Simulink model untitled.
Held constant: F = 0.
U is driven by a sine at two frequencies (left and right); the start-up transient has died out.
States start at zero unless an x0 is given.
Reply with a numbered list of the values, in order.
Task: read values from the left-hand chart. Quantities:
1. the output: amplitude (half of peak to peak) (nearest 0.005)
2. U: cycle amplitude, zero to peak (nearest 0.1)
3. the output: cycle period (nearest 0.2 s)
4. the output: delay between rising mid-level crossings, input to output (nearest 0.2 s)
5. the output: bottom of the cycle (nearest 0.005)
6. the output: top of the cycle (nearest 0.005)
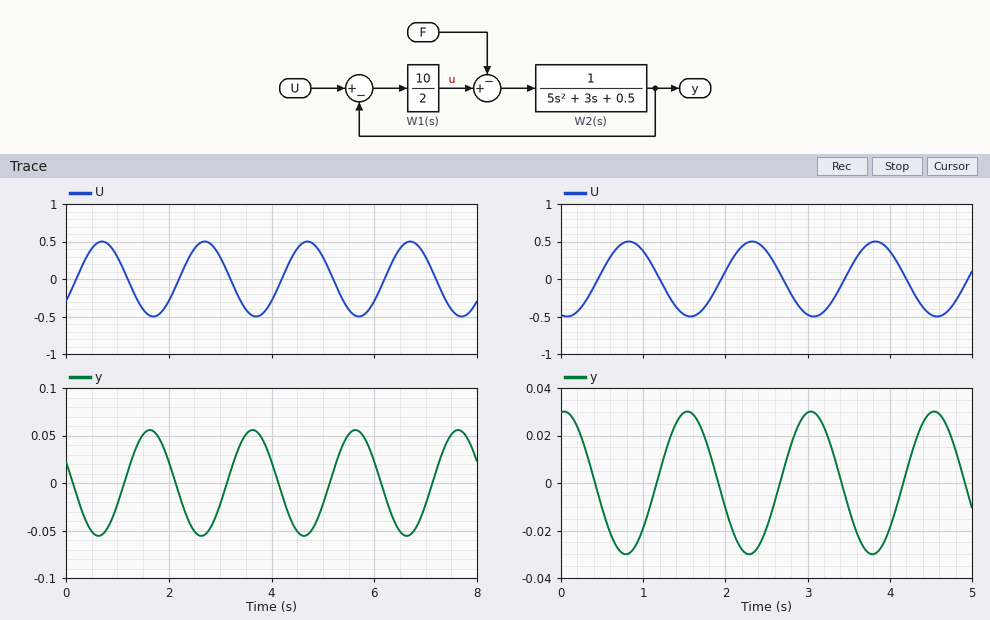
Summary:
1. 0.055
2. 0.5
3. 2.0 s
4. 1.0 s
5. -0.055
6. 0.055
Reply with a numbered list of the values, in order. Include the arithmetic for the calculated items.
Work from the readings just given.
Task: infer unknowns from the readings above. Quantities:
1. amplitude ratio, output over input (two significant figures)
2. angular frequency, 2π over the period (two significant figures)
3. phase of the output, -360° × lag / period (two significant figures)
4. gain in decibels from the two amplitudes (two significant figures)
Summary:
1. 0.055 / 0.5 = 0.11
2. 2π / 2 = 3.1 rad/s
3. -360 × 1 / 2 = -180°
4. 20 log10(0.055 / 0.5) = -19 dB
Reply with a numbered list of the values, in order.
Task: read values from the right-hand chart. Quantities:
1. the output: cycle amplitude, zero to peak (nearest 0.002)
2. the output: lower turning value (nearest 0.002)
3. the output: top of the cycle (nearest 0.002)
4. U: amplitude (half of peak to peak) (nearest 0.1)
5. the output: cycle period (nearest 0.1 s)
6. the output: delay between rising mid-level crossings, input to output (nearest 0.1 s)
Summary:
1. 0.030
2. -0.030
3. 0.030
4. 0.5
5. 1.5 s
6. 0.7 s
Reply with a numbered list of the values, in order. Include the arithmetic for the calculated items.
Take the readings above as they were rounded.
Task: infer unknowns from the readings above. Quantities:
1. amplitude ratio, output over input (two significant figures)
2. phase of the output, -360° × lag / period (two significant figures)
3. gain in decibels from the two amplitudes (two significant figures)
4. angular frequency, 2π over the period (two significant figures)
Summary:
1. 0.03 / 0.5 = 0.060
2. -360 × 0.7 / 1.5 = -170°
3. 20 log10(0.03 / 0.5) = -24 dB
4. 2π / 1.5 = 4.2 rad/s
